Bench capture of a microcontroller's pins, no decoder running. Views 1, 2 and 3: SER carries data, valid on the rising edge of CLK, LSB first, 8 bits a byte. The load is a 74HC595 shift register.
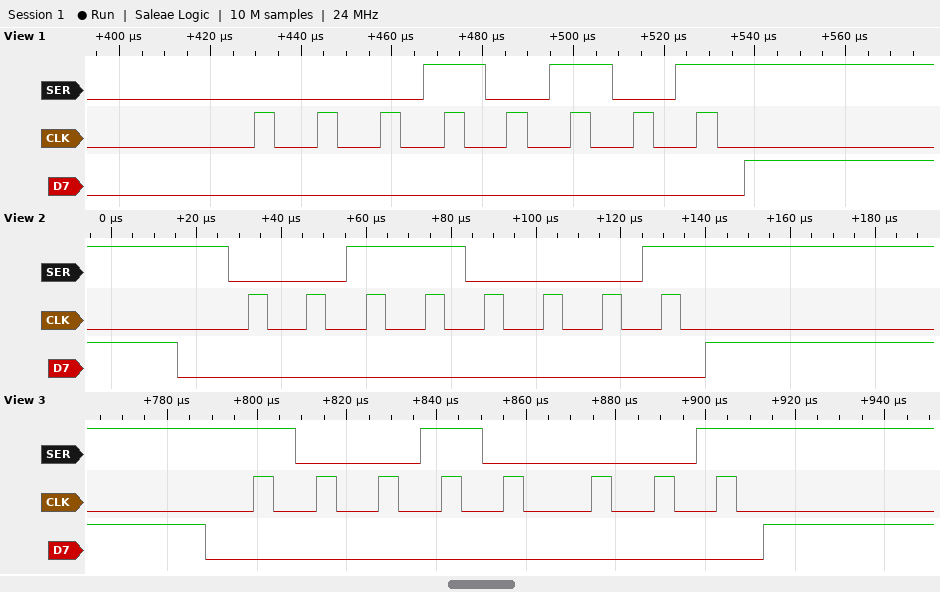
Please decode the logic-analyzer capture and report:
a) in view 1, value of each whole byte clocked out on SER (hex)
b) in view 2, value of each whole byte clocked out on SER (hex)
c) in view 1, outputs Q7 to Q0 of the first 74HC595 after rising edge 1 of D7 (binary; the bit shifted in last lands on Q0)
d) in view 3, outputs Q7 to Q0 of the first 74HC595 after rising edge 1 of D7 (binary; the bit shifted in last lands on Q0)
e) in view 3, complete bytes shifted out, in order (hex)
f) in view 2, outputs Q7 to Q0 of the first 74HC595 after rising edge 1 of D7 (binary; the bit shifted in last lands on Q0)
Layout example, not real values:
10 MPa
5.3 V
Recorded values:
A8
0x8C
00010101
10010001
0x89
00110001
